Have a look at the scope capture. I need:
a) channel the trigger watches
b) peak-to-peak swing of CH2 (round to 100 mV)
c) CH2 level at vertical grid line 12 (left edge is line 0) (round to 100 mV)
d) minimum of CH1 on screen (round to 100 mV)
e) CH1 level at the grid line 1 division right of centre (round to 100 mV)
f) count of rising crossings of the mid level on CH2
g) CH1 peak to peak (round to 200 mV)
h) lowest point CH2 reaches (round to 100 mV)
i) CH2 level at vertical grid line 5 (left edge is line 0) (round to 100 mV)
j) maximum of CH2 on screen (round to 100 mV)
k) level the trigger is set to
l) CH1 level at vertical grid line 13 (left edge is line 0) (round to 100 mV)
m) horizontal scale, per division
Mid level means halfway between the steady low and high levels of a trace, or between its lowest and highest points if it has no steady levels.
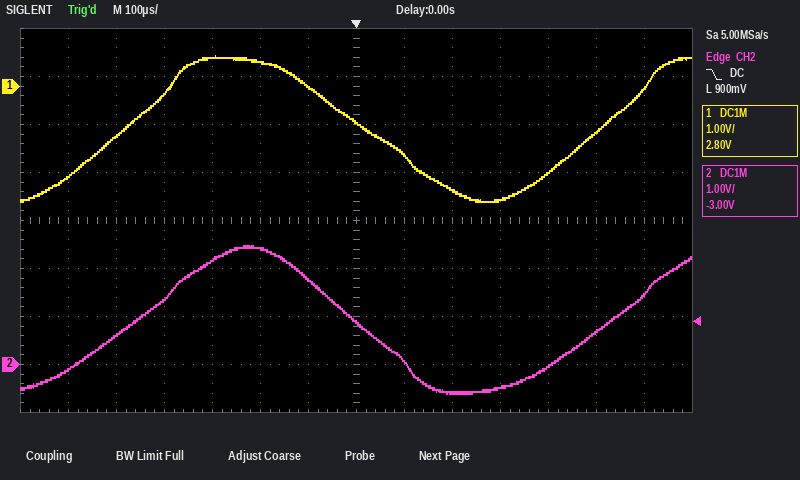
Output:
CH2
3.1 V
700 mV
-2.4 V
-1.4 V
2
3.0 V
-600 mV
2.4 V
2.5 V
900 mV
-100 mV
100 µs
